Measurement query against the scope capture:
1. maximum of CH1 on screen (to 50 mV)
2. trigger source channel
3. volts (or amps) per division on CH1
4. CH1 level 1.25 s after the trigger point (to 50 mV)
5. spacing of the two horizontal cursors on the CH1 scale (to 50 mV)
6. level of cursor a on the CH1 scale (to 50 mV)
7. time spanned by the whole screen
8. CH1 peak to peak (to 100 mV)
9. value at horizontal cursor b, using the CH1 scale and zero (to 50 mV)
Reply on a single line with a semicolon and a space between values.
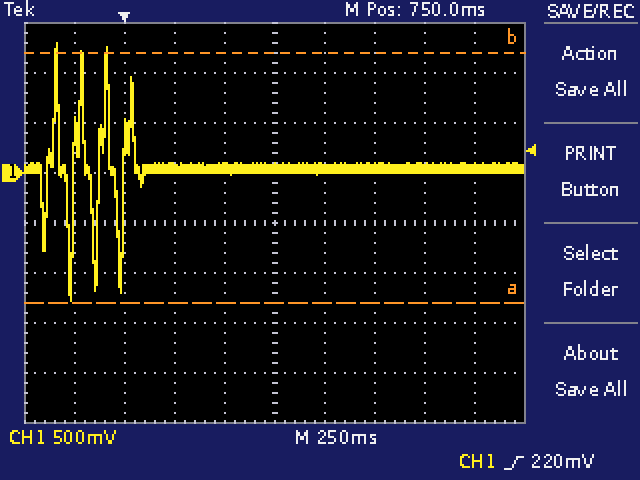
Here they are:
1.30 V; CH1; 500 mV; 50 mV; 2.50 V; -1.30 V; 2.5 s; 2.60 V; 1.20 V
